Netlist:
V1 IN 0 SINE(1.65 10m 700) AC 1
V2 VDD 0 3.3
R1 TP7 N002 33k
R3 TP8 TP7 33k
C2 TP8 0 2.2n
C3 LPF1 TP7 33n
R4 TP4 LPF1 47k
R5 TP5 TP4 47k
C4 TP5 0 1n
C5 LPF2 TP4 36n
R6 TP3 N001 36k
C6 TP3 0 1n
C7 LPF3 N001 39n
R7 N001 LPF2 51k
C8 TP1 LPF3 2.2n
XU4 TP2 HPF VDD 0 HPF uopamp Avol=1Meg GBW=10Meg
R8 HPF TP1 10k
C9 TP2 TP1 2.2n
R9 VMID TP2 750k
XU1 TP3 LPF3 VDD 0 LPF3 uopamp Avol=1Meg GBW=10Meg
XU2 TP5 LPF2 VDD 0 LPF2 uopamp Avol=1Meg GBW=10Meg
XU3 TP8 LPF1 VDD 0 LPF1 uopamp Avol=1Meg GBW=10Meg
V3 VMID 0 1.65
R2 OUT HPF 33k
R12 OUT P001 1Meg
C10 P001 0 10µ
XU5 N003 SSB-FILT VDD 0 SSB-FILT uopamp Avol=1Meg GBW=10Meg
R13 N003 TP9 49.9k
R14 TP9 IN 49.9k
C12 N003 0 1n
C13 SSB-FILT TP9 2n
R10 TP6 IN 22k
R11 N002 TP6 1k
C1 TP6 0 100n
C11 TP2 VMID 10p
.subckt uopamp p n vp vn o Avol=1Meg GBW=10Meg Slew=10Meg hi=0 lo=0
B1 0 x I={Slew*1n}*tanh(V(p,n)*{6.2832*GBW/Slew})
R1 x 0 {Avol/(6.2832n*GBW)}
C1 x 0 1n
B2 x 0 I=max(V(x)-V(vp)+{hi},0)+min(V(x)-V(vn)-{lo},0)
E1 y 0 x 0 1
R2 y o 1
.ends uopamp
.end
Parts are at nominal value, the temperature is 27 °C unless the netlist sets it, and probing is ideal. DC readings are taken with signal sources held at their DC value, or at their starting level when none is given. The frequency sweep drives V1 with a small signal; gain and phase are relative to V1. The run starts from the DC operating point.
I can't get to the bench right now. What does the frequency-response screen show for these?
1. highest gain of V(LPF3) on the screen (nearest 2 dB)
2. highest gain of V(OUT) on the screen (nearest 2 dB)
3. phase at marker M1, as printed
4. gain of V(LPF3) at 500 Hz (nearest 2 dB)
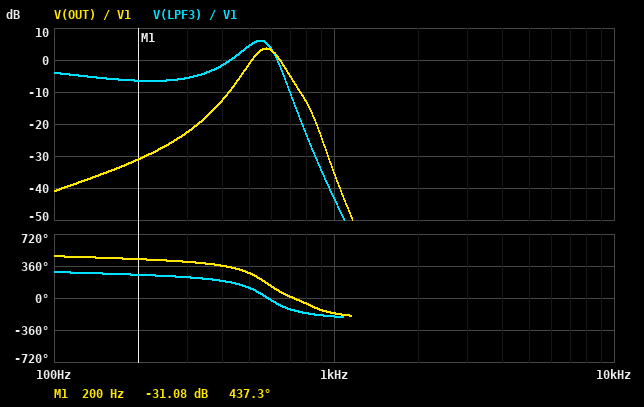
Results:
6 dB
4 dB
437.3 deg
4 dB
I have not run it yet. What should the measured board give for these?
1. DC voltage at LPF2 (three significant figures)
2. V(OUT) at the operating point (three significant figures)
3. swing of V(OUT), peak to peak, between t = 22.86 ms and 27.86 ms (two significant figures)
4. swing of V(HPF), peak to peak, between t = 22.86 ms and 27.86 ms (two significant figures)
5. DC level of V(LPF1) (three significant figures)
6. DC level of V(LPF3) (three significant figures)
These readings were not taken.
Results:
1.65 V
1.65 V
11 mV
11 mV
1.65 V
1.65 V
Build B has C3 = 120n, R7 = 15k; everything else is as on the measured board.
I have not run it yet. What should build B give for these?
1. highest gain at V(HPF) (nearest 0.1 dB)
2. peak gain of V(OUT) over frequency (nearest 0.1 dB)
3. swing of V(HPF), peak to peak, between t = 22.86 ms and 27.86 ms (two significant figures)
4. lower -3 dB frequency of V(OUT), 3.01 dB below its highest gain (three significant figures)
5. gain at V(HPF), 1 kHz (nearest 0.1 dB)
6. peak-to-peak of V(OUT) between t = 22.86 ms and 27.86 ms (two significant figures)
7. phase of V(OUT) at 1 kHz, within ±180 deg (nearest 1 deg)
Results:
-17.0 dB
-17.3 dB
1.9 mV
273 Hz
-33.3 dB
1.8 mV
-89 deg
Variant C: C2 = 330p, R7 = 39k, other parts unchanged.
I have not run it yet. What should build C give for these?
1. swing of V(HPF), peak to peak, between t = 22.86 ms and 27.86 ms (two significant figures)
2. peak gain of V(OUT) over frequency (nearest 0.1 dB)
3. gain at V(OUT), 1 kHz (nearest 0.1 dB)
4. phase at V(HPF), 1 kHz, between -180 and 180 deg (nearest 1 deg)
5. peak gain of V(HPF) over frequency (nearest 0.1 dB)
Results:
22 mV
1.1 dB
-18.4 dB
-30 deg
1.4 dB
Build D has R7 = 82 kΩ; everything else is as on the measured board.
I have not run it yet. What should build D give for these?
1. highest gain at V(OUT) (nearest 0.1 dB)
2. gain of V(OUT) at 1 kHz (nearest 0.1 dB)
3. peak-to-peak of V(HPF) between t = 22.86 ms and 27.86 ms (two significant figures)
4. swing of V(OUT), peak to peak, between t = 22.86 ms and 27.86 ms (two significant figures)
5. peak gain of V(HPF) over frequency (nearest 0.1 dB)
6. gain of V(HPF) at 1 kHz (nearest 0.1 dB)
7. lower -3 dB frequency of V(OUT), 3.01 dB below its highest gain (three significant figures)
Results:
-0.7 dB
-40.7 dB
4.6 mV
4.4 mV
-0.4 dB
-40.5 dB
449 Hz
